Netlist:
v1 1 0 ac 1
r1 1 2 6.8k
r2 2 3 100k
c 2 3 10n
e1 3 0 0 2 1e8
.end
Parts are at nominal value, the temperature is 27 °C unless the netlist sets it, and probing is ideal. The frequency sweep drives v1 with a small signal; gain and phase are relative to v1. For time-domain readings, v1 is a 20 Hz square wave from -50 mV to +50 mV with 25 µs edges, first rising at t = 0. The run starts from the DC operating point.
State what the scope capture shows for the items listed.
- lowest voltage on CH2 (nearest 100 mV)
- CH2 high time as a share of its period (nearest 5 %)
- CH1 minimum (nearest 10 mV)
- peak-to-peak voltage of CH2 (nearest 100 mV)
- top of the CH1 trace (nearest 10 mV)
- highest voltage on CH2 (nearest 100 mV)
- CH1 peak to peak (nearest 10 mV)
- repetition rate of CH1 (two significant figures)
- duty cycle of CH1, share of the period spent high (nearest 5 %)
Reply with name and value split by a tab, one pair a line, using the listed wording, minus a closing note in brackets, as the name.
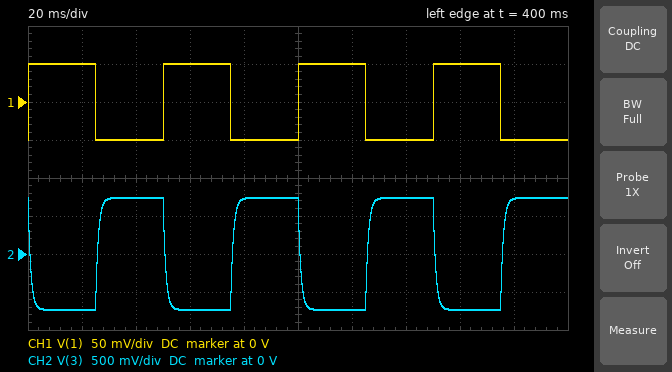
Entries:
lowest voltage on CH2	-700 mV
CH2 high time as a share of its period	50 %
CH1 minimum	-50 mV
peak-to-peak voltage of CH2	1.5 V
top of the CH1 trace	50 mV
highest voltage on CH2	700 mV
CH1 peak to peak	100 mV
repetition rate of CH1	20 Hz
duty cycle of CH1, share of the period spent high	50 %
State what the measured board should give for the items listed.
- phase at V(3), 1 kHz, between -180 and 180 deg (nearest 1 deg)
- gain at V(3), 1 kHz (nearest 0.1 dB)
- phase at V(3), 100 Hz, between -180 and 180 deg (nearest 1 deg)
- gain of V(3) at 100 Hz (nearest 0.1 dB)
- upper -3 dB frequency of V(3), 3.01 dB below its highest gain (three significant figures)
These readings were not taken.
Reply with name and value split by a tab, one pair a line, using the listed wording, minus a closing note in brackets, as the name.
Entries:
phase at V(3), 1 kHz, between -180 and 180 deg	99 deg
gain at V(3), 1 kHz	7.3 dB
phase at V(3), 100 Hz, between -180 and 180 deg	148 deg
gain of V(3) at 100 Hz	21.9 dB
upper -3 dB frequency of V(3), 3.01 dB below its highest gain	159 Hz
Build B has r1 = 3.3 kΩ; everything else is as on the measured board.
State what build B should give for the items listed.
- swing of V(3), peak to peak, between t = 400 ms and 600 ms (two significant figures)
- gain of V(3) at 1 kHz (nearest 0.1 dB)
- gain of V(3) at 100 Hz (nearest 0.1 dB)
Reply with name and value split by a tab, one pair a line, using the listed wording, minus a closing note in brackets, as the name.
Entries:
swing of V(3), peak to peak, between t = 400 ms and 600 ms	3.0 V
gain of V(3) at 1 kHz	13.6 dB
gain of V(3) at 100 Hz	28.2 dB
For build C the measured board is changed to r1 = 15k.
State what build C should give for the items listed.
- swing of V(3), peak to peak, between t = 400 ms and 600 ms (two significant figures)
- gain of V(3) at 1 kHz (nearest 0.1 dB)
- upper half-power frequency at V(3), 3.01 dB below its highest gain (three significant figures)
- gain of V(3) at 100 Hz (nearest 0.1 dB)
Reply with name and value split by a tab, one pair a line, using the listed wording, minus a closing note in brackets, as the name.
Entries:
swing of V(3), peak to peak, between t = 400 ms and 600 ms	670 mV
gain of V(3) at 1 kHz	0.4 dB
upper half-power frequency at V(3), 3.01 dB below its highest gain	159 Hz
gain of V(3) at 100 Hz	15.0 dB
